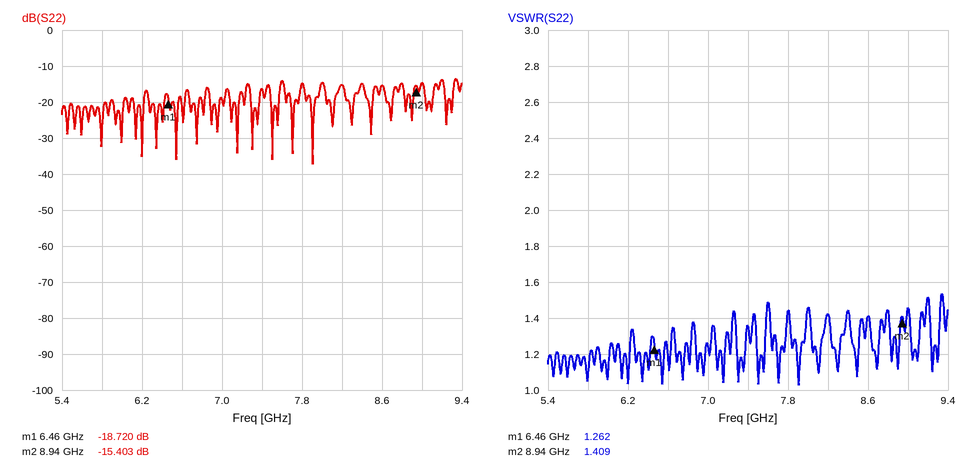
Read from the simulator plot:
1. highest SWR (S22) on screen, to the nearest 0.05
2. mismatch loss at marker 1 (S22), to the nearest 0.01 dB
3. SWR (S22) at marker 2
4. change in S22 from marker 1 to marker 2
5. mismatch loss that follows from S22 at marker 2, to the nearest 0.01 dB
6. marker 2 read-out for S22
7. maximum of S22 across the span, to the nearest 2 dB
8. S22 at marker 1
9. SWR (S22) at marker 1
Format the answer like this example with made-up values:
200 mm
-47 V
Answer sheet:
1.55
0.06 dB
1.409
3.317 dB
0.13 dB
-15.403 dB
-14 dB
-18.720 dB
1.262
